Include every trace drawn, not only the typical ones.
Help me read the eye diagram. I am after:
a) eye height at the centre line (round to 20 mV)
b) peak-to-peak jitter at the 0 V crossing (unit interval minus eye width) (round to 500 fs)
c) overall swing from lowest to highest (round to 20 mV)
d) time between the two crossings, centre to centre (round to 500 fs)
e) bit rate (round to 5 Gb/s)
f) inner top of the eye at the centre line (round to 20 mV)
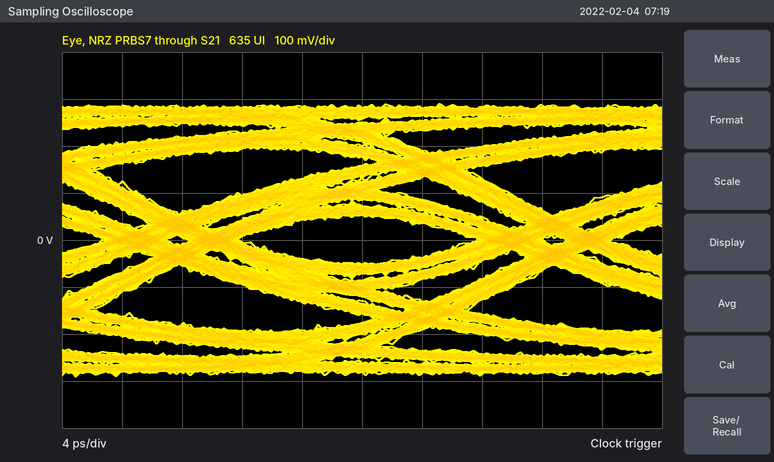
100 mV
9.0 ps
580 mV
25.0 ps
40 Gb/s
60 mV
